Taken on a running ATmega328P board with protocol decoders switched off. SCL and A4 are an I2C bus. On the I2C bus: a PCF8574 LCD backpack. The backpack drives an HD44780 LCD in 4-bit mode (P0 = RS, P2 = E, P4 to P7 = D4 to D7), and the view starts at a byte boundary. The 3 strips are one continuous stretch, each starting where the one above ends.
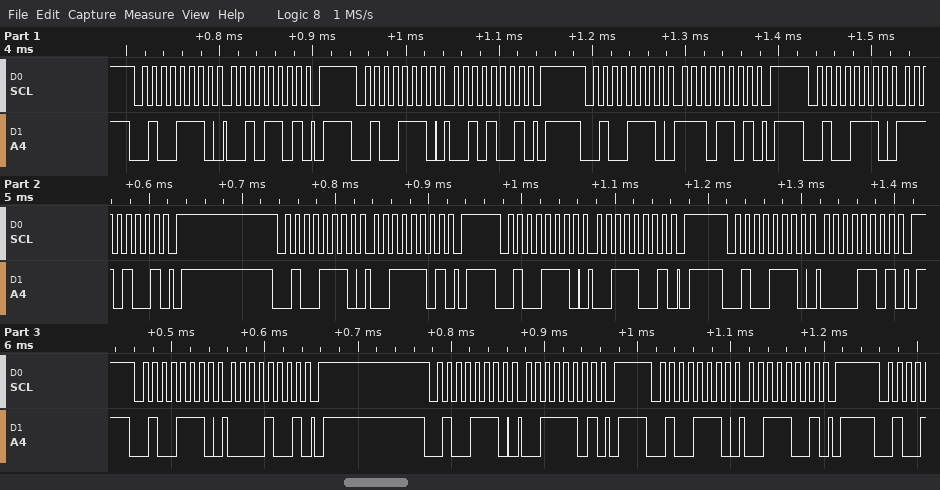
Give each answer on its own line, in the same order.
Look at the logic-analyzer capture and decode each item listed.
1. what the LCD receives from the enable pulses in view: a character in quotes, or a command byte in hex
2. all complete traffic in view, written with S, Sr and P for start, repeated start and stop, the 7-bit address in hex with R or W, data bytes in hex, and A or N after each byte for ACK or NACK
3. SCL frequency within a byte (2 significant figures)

'.' '0'
S 27W A 2D A P S 27W A 29 A P S 27W A ED A P S 27W A E9 A P S 27W A 3D A P S 27W A 39 A P S 27W A 0D A P S 27W A 09 A P S 27W A 3D A P S 27W A 39 A P
100 kHz
